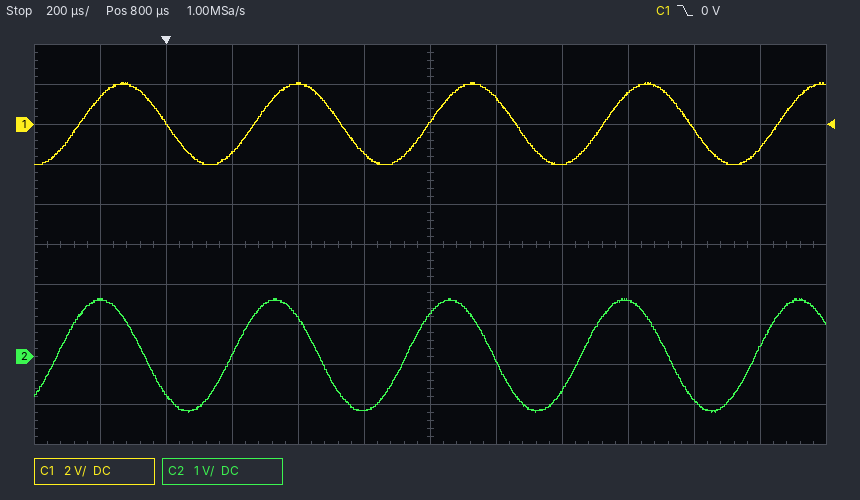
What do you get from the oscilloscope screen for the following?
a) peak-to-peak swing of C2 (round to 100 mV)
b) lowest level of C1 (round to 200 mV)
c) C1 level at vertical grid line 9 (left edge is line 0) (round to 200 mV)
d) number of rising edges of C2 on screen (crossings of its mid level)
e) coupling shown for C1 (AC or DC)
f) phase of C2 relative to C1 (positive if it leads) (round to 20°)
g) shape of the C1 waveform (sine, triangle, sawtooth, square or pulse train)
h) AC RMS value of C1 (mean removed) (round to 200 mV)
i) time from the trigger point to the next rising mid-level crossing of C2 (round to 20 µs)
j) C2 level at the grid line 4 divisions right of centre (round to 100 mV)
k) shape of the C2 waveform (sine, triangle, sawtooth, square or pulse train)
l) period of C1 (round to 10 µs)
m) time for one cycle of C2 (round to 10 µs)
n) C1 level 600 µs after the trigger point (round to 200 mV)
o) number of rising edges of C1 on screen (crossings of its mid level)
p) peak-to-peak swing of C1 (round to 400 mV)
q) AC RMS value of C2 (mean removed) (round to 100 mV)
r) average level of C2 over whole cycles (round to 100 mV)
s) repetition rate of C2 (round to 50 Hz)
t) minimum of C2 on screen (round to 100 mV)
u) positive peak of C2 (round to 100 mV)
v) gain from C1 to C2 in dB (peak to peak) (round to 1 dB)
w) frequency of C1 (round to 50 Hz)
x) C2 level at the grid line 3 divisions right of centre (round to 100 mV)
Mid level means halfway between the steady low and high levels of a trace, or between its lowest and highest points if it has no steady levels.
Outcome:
2.8 V
-2.0 V
1.6 V
5
DC
+40°
sine
1.4 V
200 µs
-1.1 V
sine
530 µs
530 µs
-1.4 V
5
4.0 V
1.0 V
0.0 V
1.90 kHz
-1.4 V
1.4 V
-3 dB
1.90 kHz
1.4 V
